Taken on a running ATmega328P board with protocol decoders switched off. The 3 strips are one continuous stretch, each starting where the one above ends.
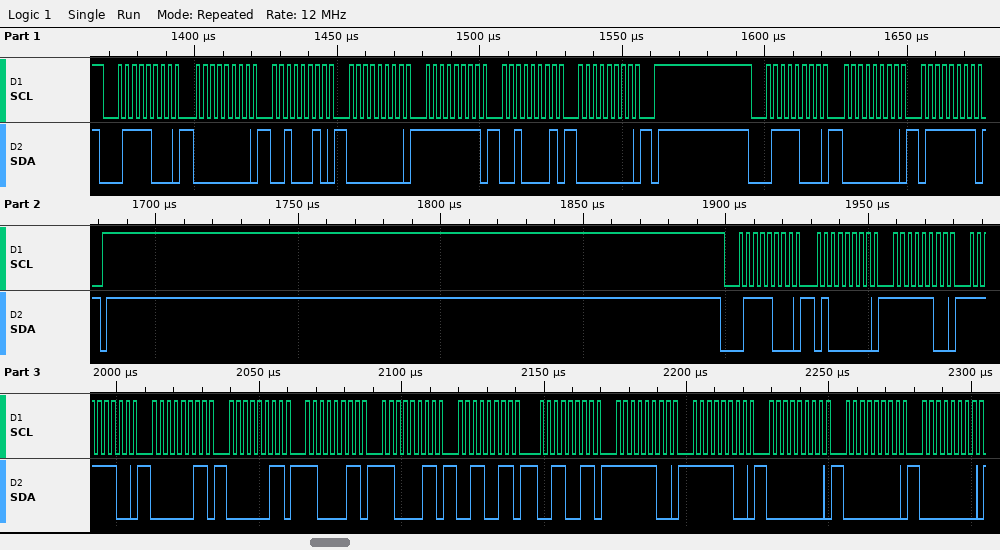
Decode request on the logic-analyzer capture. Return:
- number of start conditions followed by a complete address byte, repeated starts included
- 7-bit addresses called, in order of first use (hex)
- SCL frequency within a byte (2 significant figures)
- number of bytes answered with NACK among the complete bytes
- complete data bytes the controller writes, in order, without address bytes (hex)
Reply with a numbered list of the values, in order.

1. 3
2. 0x3C
3. 400 kHz
4. 0
5. 00 22 00 FF 21 00 00 7F 40 FC FC 03 03 C3 C3 33 33 FC FC 00 00 00
